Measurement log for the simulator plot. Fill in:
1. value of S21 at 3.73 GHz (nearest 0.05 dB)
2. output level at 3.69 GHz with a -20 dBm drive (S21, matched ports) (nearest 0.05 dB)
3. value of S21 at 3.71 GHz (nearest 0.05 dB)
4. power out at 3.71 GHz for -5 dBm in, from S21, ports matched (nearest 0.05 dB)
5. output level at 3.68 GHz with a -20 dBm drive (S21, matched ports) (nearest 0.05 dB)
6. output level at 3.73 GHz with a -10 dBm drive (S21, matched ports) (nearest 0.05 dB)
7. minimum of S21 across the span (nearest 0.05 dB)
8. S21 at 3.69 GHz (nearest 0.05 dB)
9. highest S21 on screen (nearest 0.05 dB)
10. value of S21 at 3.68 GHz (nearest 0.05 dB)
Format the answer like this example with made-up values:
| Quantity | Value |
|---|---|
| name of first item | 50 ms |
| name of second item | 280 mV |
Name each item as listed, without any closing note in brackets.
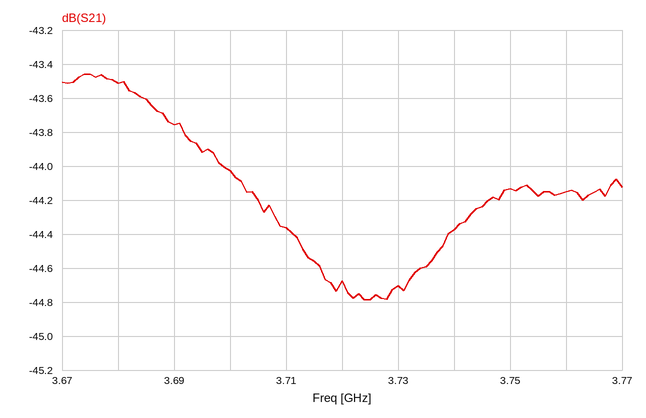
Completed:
| Quantity | Value |
|---|---|
| value of S21 at 3.73 GHz | -44.70 dB |
| output level at 3.69 GHz with a -20 dBm drive (S21, matched ports) | -63.75 dBm |
| value of S21 at 3.71 GHz | -44.35 dB |
| power out at 3.71 GHz for -5 dBm in, from S21, ports matched | -49.35 dBm |
| output level at 3.68 GHz with a -20 dBm drive (S21, matched ports) | -63.50 dBm |
| output level at 3.73 GHz with a -10 dBm drive (S21, matched ports) | -54.70 dBm |
| minimum of S21 across the span | -44.80 dB |
| S21 at 3.69 GHz | -43.75 dB |
| highest S21 on screen | -43.45 dB |
| value of S21 at 3.68 GHz | -43.50 dB |
